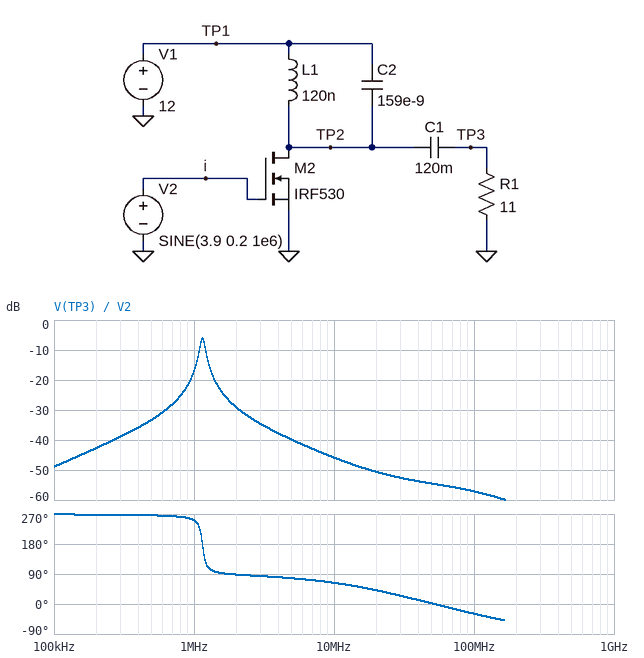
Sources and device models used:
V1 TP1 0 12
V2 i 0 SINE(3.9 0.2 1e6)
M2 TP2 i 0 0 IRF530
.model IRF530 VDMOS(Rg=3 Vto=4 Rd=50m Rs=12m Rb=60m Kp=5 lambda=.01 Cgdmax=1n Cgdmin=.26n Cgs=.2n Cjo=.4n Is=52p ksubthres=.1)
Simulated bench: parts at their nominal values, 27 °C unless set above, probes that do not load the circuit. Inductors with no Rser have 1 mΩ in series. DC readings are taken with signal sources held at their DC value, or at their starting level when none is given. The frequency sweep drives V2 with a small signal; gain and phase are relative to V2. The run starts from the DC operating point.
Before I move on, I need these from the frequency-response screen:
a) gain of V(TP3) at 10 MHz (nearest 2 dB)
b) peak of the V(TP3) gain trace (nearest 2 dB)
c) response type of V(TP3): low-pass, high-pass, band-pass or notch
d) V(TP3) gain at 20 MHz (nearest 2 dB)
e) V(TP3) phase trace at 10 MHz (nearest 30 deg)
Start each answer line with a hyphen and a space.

- -46 dB
- -6 dB
- band-pass
- -50 dB
- 60 deg
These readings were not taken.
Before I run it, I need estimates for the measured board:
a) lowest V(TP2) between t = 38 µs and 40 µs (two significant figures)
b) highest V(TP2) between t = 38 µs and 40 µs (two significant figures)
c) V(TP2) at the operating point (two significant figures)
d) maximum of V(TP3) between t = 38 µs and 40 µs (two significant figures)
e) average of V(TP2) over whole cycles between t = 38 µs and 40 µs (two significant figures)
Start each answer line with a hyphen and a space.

- 12 V
- 12 V
- 12 V
- 66 mV
- 12 V
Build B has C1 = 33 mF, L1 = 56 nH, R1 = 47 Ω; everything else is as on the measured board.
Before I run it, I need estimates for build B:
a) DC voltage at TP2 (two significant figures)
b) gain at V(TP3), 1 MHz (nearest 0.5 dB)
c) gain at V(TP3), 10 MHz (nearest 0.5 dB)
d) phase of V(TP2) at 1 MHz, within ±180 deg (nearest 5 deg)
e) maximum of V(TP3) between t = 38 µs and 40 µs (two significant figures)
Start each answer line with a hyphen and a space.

- 12 V
- -32.0 dB
- -45.5 dB
- -95 deg
- 27 mV
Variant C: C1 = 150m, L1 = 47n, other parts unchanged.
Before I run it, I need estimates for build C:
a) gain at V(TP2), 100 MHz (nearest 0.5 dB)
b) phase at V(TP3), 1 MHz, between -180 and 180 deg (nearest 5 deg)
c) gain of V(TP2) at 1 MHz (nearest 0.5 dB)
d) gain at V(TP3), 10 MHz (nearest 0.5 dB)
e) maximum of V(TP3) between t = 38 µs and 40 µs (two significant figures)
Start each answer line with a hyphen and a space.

- -57.0 dB
- -95 deg
- -34.0 dB
- -45.5 dB
- 39 mV
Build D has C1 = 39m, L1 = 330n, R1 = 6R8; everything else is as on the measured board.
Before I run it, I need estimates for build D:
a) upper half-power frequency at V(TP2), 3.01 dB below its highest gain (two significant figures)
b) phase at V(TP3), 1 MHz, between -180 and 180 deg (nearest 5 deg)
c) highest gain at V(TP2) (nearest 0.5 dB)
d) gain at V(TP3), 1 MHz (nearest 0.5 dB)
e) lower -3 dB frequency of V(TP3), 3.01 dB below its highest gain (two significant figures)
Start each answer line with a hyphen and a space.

- 770 kHz
- 105 deg
- -10.0 dB
- -21.0 dB
- 620 kHz
